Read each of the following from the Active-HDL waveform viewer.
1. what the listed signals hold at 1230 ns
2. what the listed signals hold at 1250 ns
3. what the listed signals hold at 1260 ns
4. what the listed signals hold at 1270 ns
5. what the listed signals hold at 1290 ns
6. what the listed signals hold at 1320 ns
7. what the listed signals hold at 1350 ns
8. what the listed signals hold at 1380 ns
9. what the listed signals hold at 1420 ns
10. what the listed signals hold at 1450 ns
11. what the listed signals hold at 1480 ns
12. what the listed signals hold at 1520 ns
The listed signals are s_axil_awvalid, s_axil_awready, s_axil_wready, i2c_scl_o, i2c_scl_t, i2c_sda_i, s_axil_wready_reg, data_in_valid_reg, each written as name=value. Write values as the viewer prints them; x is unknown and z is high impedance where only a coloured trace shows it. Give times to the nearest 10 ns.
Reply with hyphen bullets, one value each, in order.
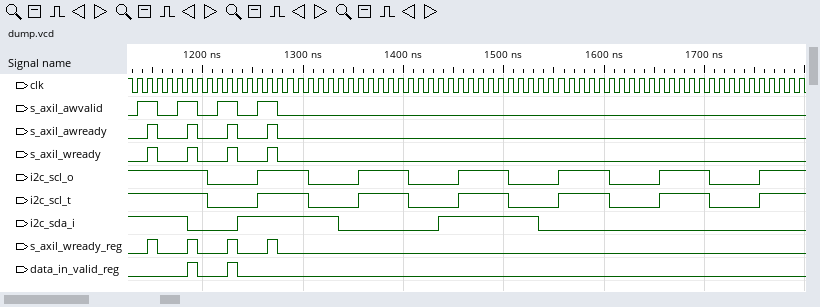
- s_axil_awvalid=1, s_axil_awready=1, s_axil_wready=1, i2c_scl_o=0, i2c_scl_t=0, i2c_sda_i=0, s_axil_wready_reg=1, data_in_valid_reg=1
- s_axil_awvalid=0, s_axil_awready=0, s_axil_wready=0, i2c_scl_o=0, i2c_scl_t=0, i2c_sda_i=1, s_axil_wready_reg=0, data_in_valid_reg=0
- s_axil_awvalid=1, s_axil_awready=0, s_axil_wready=0, i2c_scl_o=1, i2c_scl_t=1, i2c_sda_i=1, s_axil_wready_reg=0, data_in_valid_reg=0
- s_axil_awvalid=1, s_axil_awready=1, s_axil_wready=1, i2c_scl_o=1, i2c_scl_t=1, i2c_sda_i=1, s_axil_wready_reg=1, data_in_valid_reg=0
- s_axil_awvalid=0, s_axil_awready=0, s_axil_wready=0, i2c_scl_o=1, i2c_scl_t=1, i2c_sda_i=1, s_axil_wready_reg=0, data_in_valid_reg=0
- s_axil_awvalid=0, s_axil_awready=0, s_axil_wready=0, i2c_scl_o=0, i2c_scl_t=0, i2c_sda_i=1, s_axil_wready_reg=0, data_in_valid_reg=0
- s_axil_awvalid=0, s_axil_awready=0, s_axil_wready=0, i2c_scl_o=0, i2c_scl_t=0, i2c_sda_i=0, s_axil_wready_reg=0, data_in_valid_reg=0
- s_axil_awvalid=0, s_axil_awready=0, s_axil_wready=0, i2c_scl_o=1, i2c_scl_t=1, i2c_sda_i=0, s_axil_wready_reg=0, data_in_valid_reg=0
- s_axil_awvalid=0, s_axil_awready=0, s_axil_wready=0, i2c_scl_o=0, i2c_scl_t=0, i2c_sda_i=0, s_axil_wready_reg=0, data_in_valid_reg=0
- s_axil_awvalid=0, s_axil_awready=0, s_axil_wready=0, i2c_scl_o=0, i2c_scl_t=0, i2c_sda_i=1, s_axil_wready_reg=0, data_in_valid_reg=0
- s_axil_awvalid=0, s_axil_awready=0, s_axil_wready=0, i2c_scl_o=1, i2c_scl_t=1, i2c_sda_i=1, s_axil_wready_reg=0, data_in_valid_reg=0
- s_axil_awvalid=0, s_axil_awready=0, s_axil_wready=0, i2c_scl_o=0, i2c_scl_t=0, i2c_sda_i=1, s_axil_wready_reg=0, data_in_valid_reg=0
